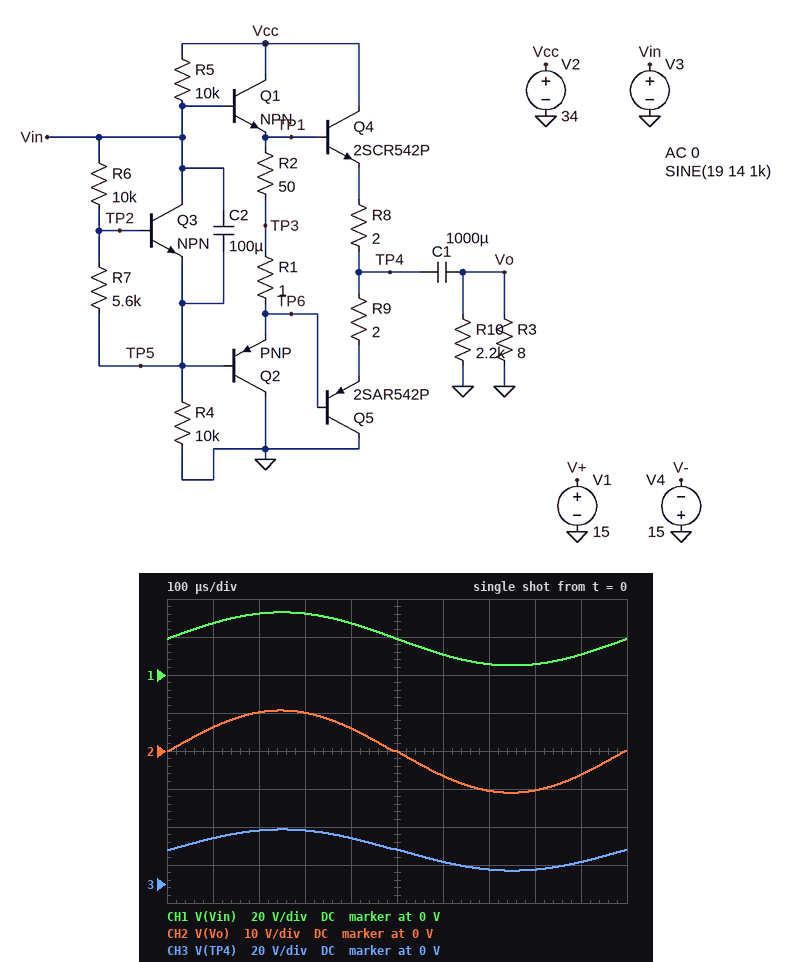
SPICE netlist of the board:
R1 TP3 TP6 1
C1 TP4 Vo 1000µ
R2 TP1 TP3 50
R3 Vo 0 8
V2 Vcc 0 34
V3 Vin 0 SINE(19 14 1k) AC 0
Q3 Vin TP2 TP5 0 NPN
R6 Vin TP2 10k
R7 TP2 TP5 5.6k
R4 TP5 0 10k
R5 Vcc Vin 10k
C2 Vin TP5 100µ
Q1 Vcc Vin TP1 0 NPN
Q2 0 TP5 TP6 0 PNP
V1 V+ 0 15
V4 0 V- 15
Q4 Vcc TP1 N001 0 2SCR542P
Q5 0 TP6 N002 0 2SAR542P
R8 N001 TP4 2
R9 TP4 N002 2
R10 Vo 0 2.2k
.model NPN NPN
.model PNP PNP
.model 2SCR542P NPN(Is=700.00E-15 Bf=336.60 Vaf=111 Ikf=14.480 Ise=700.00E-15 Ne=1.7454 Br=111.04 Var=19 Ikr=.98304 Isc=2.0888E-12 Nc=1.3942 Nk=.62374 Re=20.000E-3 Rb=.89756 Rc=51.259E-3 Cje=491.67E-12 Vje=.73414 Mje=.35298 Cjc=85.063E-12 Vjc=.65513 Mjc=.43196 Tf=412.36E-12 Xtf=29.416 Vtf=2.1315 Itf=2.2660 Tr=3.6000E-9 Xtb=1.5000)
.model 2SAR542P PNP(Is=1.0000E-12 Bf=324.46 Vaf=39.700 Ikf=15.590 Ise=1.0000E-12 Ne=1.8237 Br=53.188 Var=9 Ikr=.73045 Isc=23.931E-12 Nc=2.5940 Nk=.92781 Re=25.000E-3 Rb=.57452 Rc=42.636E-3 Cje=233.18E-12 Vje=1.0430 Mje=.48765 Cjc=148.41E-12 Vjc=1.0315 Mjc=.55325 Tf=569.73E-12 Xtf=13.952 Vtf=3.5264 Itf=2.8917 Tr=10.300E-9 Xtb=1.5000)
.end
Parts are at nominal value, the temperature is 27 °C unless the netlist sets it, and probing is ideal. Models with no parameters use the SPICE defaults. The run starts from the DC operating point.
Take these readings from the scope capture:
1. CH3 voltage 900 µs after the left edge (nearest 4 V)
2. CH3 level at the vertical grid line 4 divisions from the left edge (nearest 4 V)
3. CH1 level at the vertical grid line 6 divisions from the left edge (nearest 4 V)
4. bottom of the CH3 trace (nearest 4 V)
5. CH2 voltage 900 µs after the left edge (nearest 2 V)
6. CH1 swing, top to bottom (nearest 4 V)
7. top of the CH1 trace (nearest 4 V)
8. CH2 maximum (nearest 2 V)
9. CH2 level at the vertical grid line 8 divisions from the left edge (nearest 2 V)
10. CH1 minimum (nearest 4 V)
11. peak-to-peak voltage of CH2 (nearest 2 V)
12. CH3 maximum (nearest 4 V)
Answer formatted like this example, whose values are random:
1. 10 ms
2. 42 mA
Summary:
1. 12 V
2. 24 V
3. 12 V
4. 8 V
5. -6 V
6. 28 V
7. 32 V
8. 10 V
9. -10 V
10. 4 V
11. 22 V
12. 28 V
